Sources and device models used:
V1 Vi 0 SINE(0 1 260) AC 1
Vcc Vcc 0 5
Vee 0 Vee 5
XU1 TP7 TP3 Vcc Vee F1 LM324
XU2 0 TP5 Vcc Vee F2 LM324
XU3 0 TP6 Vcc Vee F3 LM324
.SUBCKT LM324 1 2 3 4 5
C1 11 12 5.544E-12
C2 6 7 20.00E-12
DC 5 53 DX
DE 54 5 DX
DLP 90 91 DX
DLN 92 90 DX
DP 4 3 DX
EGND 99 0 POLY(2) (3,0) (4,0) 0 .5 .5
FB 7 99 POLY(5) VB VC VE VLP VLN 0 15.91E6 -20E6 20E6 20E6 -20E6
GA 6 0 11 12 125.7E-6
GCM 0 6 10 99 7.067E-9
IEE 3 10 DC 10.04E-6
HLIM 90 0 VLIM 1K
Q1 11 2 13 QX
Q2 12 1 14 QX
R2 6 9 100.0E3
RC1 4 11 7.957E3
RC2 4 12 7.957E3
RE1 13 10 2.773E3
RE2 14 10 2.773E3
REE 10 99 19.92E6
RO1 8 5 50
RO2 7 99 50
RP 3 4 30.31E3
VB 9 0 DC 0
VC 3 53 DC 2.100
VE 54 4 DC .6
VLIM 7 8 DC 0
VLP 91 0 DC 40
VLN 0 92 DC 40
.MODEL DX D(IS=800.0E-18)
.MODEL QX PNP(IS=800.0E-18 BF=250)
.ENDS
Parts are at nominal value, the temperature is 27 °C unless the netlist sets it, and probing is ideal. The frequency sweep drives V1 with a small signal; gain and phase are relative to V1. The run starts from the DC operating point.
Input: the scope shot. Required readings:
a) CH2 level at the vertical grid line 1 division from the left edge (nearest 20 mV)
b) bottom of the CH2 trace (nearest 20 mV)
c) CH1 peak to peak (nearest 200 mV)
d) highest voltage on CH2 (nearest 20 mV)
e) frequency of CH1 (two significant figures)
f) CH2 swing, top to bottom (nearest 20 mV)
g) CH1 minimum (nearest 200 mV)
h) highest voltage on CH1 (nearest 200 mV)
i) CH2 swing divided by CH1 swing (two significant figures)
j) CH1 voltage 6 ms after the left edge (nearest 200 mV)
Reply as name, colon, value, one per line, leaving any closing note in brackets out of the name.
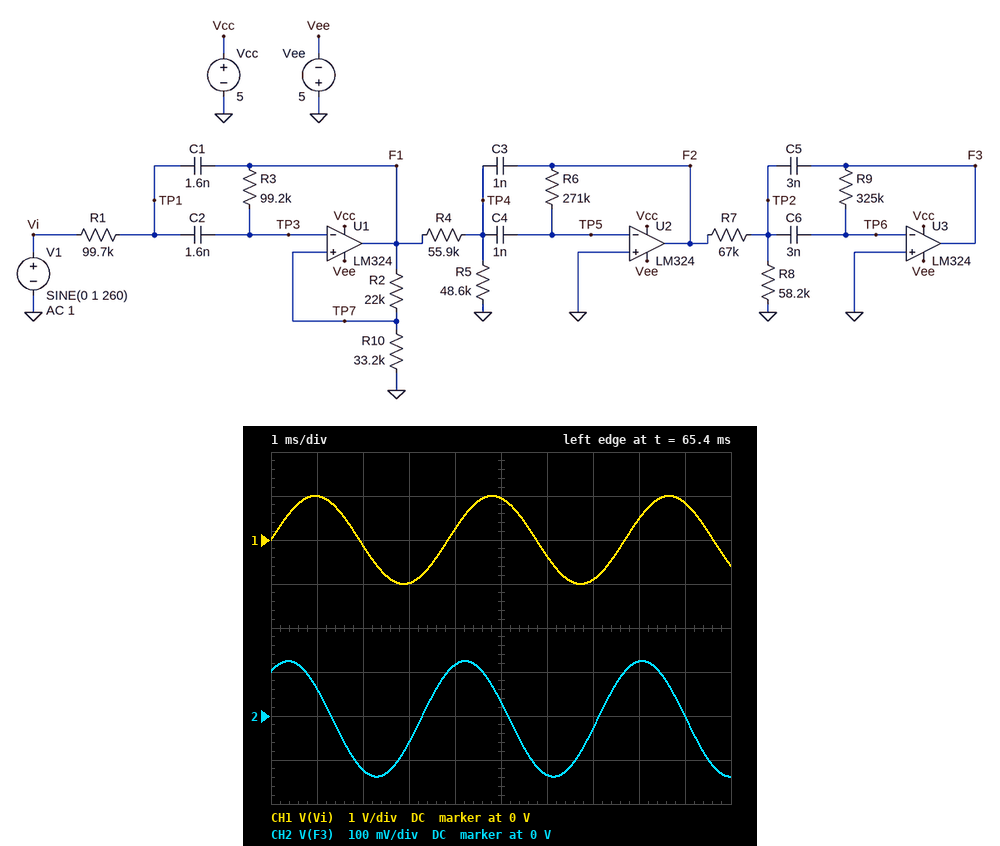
CH2 level at the vertical grid line 1 division from the left edge: 60 mV
bottom of the CH2 trace: -140 mV
CH1 peak to peak: 2.0 V
highest voltage on CH2: 120 mV
frequency of CH1: 260 Hz
CH2 swing, top to bottom: 260 mV
CH1 minimum: -1.0 V
highest voltage on CH1: 1.0 V
CH2 swing divided by CH1 swing: 0.13
CH1 voltage 6 ms after the left edge: -400 mV
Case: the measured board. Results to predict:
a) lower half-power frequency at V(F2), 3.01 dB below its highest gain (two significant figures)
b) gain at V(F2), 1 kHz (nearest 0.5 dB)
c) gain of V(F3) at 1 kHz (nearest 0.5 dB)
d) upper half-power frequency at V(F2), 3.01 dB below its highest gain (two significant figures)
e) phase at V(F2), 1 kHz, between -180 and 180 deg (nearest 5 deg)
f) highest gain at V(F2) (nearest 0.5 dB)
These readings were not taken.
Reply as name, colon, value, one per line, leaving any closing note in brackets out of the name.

lower half-power frequency at V(F2), 3.01 dB below its highest gain: 890 Hz
gain at V(F2), 1 kHz: 14.0 dB
gain of V(F3) at 1 kHz: 14.0 dB
upper half-power frequency at V(F2), 3.01 dB below its highest gain: 2.0 kHz
phase at V(F2), 1 kHz, between -180 and 180 deg: 65 deg
highest gain at V(F2): 14.5 dB
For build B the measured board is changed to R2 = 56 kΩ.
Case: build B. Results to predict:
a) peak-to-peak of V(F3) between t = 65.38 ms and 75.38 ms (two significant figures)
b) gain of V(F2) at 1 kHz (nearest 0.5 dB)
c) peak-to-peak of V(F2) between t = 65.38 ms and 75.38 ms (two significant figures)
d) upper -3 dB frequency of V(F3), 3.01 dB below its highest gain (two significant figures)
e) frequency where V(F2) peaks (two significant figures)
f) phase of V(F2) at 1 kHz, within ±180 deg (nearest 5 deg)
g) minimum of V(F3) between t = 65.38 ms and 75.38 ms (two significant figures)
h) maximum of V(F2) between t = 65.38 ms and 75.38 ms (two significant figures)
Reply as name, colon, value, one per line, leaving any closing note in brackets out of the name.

peak-to-peak of V(F3) between t = 65.38 ms and 75.38 ms: 160 mV
gain of V(F2) at 1 kHz: 1.0 dB
peak-to-peak of V(F2) between t = 65.38 ms and 75.38 ms: 170 mV
upper -3 dB frequency of V(F3), 3.01 dB below its highest gain: 2.0 kHz
frequency where V(F2) peaks: 1.7 kHz
phase of V(F2) at 1 kHz, within ±180 deg: 65 deg
minimum of V(F3) between t = 65.38 ms and 75.38 ms: -85 mV
maximum of V(F2) between t = 65.38 ms and 75.38 ms: 81 mV
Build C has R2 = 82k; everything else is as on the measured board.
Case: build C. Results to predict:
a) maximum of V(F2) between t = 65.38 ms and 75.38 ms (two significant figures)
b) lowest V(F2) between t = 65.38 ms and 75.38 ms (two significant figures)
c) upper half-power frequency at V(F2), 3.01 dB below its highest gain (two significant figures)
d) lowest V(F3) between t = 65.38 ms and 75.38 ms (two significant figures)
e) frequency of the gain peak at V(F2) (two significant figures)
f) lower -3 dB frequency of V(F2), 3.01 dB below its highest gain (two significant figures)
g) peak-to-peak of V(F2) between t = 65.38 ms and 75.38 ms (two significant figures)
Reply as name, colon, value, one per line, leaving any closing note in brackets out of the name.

maximum of V(F2) between t = 65.38 ms and 75.38 ms: 69 mV
lowest V(F2) between t = 65.38 ms and 75.38 ms: -80 mV
upper half-power frequency at V(F2), 3.01 dB below its highest gain: 2.3 kHz
lowest V(F3) between t = 65.38 ms and 75.38 ms: -74 mV
frequency of the gain peak at V(F2): 1.8 kHz
lower -3 dB frequency of V(F2), 3.01 dB below its highest gain: 1.2 kHz
peak-to-peak of V(F2) between t = 65.38 ms and 75.38 ms: 150 mV
